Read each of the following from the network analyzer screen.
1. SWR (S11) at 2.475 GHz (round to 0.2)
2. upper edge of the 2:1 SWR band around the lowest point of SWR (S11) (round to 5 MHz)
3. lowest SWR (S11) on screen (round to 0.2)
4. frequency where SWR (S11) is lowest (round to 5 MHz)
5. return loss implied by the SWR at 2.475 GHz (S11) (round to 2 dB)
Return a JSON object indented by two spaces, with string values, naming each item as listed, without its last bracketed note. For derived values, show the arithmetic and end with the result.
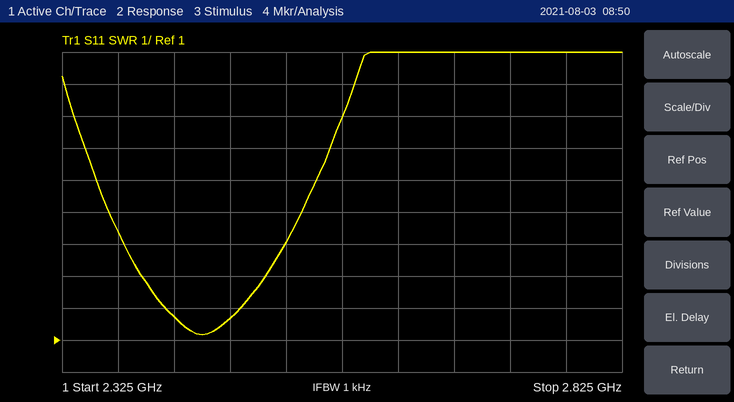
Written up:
{
  "SWR (S11) at 2.475 GHz": "1.6",
  "upper edge of the 2:1 SWR band around the lowest point of SWR (S11)": "2.485 GHz",
  "lowest SWR (S11) on screen": "1.2",
  "frequency where SWR (S11) is lowest": "2.450 GHz",
  "return loss implied by the SWR at 2.475 GHz (S11)": "−20 log10((1.6 − 1)/(1.6 + 1)) ≈ 12.7 dB, so 12 dB to the nearest 2 dB"
}
